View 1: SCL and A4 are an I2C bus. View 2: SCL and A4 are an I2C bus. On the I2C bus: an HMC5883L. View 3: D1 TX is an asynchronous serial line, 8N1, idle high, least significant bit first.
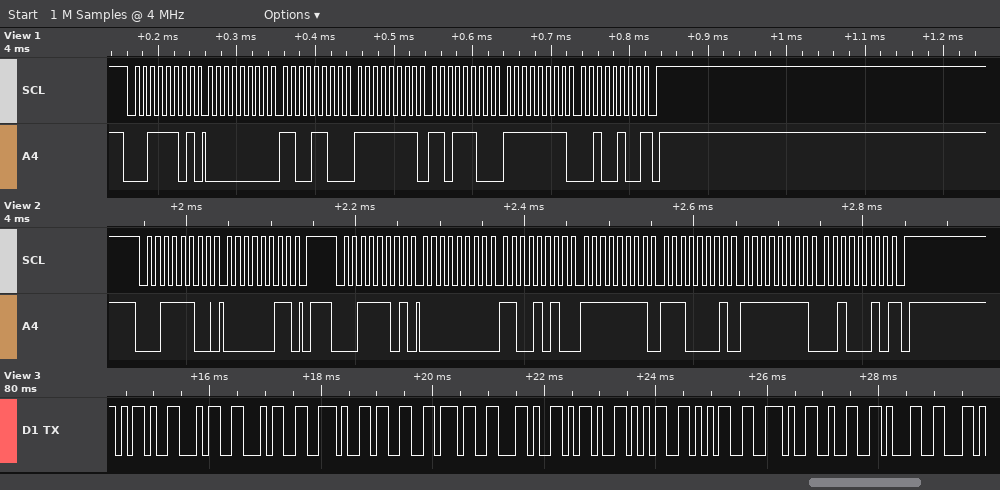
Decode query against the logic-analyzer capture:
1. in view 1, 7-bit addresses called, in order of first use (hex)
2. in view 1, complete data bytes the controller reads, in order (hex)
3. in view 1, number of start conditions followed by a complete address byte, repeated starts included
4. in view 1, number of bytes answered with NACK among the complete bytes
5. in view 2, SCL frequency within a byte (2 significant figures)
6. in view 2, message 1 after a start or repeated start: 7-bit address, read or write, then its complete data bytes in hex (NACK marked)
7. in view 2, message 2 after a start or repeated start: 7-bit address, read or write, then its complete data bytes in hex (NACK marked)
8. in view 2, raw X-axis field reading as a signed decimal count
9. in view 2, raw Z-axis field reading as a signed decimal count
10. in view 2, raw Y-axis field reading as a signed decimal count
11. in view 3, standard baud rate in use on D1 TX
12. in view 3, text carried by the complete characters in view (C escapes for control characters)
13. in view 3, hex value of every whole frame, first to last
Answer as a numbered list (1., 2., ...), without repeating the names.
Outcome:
1. 0x1E
2. 00 CC FF DC FF 24
3. 1
4. 1
5. 100 kHz
6. 0x1E write: 03
7. 0x1E read: 00 CA FF E1 FF 22 NACK
8. 202
9. -31
10. -222
11. 9600 baud
12. "-44.37,-55.21"
13. 2D 34 34 2E 33 37 2C 2D 35 35 2E 32 31
